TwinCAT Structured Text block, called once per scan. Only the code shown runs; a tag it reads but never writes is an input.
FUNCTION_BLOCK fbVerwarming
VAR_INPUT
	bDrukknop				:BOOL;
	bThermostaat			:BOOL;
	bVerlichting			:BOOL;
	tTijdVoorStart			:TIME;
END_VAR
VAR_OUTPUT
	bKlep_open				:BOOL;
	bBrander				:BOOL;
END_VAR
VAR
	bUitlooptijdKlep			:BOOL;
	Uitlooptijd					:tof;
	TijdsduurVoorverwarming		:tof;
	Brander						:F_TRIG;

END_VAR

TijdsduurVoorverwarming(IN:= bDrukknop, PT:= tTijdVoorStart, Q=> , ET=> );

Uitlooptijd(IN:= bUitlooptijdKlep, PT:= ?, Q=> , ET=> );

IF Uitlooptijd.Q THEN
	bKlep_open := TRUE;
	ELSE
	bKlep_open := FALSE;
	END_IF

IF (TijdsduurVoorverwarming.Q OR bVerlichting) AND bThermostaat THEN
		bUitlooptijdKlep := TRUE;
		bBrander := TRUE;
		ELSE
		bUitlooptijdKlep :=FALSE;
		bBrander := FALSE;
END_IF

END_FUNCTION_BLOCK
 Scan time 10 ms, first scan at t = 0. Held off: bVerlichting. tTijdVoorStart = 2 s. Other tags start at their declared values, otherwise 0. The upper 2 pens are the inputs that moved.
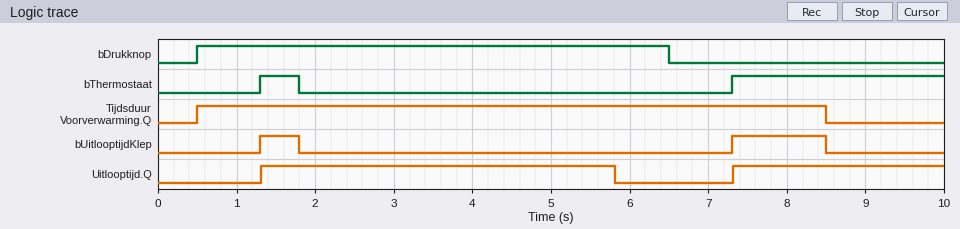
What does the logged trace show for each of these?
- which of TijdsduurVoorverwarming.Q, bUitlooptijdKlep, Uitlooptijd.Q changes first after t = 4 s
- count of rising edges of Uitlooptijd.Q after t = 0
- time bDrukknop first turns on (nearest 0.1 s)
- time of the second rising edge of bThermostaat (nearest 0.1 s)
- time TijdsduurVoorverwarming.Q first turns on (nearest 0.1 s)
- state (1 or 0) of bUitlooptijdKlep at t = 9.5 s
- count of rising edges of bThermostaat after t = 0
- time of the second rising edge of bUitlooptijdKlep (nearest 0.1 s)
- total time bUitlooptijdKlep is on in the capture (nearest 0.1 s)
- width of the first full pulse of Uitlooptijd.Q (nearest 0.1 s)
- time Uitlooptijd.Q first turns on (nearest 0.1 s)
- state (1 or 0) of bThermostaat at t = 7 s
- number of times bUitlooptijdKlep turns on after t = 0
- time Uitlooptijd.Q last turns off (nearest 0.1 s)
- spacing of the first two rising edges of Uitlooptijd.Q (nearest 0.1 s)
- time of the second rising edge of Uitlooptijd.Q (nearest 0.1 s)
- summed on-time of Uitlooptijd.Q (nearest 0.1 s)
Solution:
Uitlooptijd.Q
2
0.5 s
7.3 s
0.5 s
0
2
7.3 s
1.7 s
4.5 s
1.3 s
0
2
5.8 s
6.0 s
7.3 s
7.2 s
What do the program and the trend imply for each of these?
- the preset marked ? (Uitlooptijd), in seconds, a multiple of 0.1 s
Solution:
4.0 s
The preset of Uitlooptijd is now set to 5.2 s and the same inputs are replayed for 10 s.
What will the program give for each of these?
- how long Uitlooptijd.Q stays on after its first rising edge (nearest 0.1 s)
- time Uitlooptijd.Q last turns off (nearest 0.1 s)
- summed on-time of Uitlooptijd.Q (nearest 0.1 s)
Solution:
5.7 s
7.0 s
8.4 s
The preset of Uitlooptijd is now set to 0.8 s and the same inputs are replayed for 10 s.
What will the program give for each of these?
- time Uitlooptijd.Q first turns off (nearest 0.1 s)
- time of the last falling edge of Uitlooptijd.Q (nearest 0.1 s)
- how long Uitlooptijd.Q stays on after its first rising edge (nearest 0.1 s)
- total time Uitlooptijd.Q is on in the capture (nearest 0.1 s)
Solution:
2.6 s
9.3 s
1.3 s
3.3 s
